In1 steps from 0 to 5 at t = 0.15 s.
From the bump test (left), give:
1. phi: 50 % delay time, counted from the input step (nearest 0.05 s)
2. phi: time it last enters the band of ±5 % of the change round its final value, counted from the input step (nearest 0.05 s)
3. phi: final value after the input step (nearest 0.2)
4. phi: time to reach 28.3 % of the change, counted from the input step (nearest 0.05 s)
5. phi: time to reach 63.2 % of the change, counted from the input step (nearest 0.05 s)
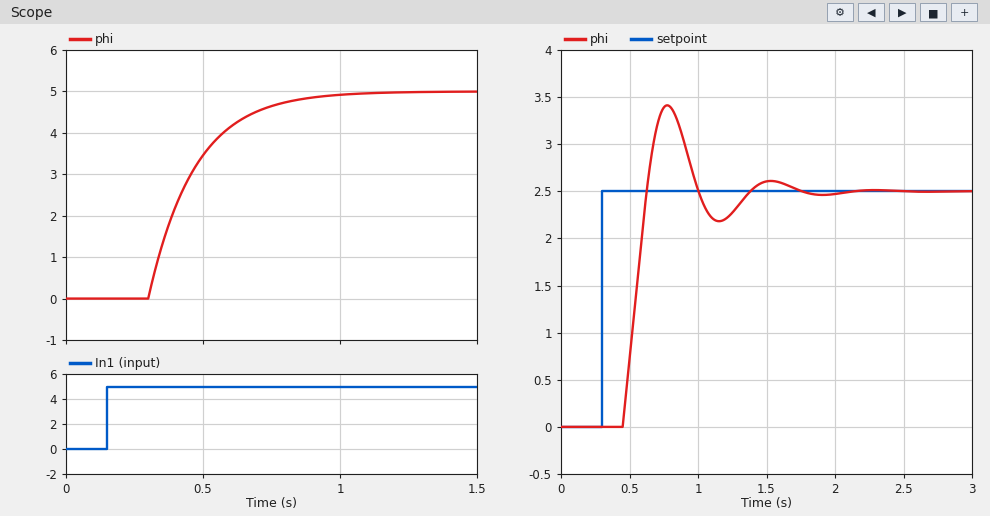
0.25 s
0.65 s
5.0
0.20 s
0.30 s
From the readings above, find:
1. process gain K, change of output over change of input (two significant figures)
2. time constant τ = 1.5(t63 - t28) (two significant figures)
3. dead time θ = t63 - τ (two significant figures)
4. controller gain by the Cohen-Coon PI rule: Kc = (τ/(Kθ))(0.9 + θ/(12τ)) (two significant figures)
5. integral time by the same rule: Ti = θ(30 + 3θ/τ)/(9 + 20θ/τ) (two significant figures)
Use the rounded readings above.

1.0
0.15 s
0.15 s
0.98
0.17 s
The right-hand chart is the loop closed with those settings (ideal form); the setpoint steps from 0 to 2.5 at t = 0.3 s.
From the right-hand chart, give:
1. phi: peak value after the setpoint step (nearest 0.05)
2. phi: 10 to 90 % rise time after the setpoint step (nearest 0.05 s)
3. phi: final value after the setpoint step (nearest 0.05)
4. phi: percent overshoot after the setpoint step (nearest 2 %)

3.40
0.15 s
2.50
36 %
